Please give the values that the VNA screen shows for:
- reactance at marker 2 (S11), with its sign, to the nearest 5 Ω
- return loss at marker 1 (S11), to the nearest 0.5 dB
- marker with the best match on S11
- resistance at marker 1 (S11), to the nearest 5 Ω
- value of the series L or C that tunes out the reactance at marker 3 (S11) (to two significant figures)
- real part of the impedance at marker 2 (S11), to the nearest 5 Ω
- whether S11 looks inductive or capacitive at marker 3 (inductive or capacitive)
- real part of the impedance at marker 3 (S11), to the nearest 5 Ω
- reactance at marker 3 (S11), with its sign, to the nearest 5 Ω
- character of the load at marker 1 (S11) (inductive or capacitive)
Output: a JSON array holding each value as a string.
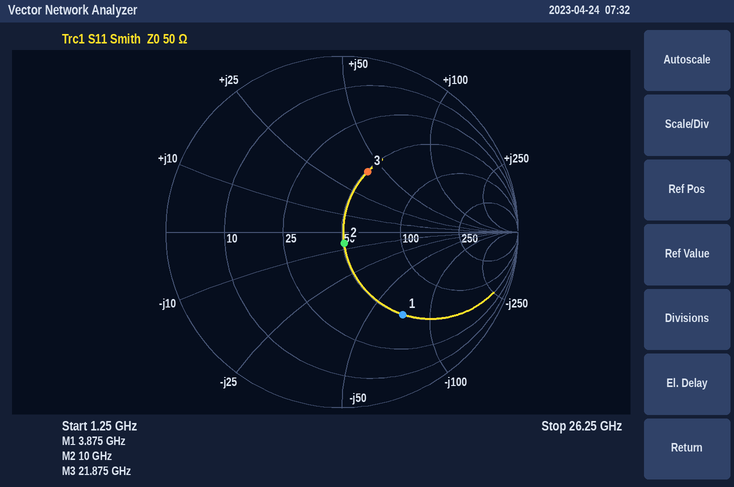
["-5 Ω", "4.5 dB", "marker 2", "50 Ω", "180 fF", "50 Ω", "inductive", "50 Ω", "+40 Ω", "capacitive"]
